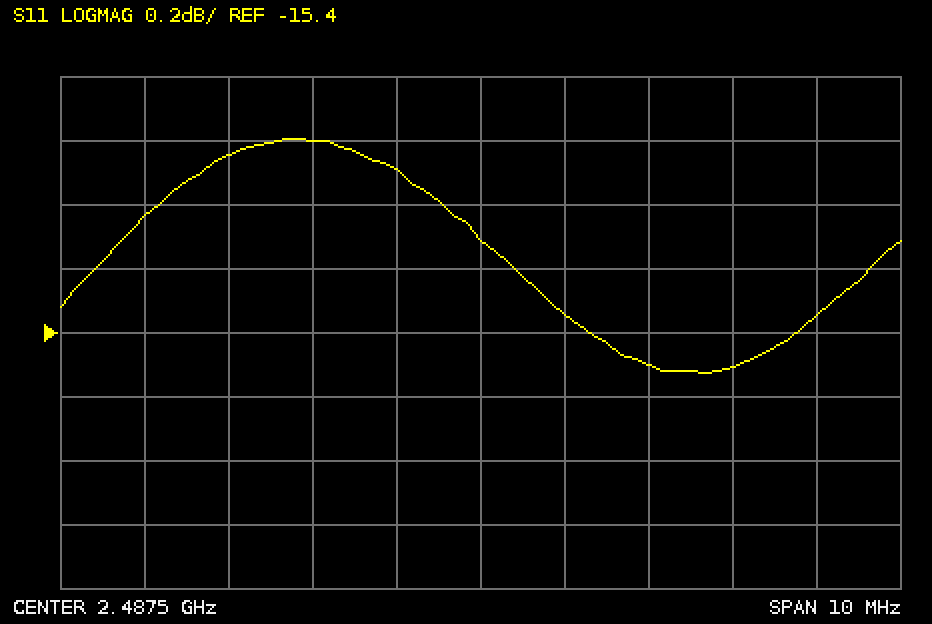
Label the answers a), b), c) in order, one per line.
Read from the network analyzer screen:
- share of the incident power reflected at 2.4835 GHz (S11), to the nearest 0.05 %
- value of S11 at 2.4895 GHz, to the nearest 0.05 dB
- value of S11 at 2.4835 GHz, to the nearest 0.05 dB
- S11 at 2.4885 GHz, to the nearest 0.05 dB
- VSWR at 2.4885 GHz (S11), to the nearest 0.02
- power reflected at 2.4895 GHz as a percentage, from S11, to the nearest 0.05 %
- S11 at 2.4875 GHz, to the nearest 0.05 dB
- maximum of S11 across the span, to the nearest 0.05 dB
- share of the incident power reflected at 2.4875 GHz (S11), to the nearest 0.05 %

a) 3.15 %
b) -15.50 dB
c) -15.05 dB
d) -15.35 dB
e) 1.42
f) 2.80 %
g) -15.10 dB
h) -14.80 dB
i) 3.10 %
